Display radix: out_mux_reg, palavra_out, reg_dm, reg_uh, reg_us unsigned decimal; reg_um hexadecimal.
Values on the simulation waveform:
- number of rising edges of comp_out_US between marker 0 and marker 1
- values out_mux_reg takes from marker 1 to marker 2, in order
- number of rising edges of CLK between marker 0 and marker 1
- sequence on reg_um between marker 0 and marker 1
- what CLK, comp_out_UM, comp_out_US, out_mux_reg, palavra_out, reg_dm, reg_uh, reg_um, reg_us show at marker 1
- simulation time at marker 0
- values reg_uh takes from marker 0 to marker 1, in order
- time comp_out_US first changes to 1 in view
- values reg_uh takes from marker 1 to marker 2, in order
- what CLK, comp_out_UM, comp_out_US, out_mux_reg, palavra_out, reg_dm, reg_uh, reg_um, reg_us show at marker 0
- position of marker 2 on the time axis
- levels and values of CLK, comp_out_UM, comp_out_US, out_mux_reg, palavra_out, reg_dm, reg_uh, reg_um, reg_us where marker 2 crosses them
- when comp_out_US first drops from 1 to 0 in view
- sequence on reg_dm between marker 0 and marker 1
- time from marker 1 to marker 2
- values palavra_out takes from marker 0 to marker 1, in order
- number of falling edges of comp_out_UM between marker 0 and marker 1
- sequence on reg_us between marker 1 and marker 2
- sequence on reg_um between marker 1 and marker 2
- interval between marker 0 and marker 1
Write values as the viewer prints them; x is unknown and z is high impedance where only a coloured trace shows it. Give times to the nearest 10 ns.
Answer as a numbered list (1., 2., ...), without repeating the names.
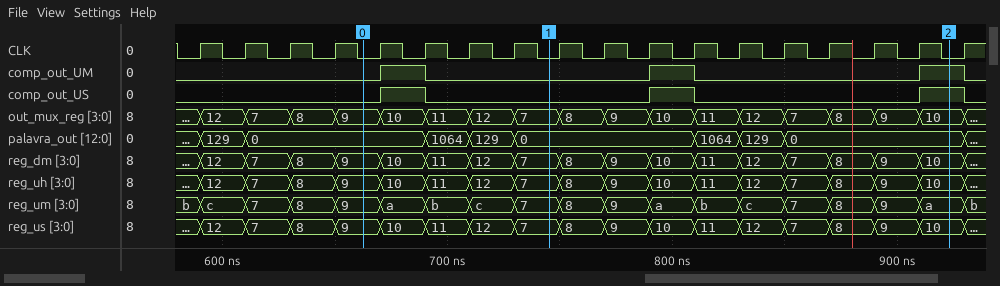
1. 1
2. 7, 8, 9, 10, 11, 12, 7, 8, 9, 10
3. 4
4. 9, a, b, c, 7
5. CLK=0, comp_out_UM=0, comp_out_US=0, out_mux_reg=7, palavra_out=0, reg_dm=7, reg_uh=7, reg_um=7, reg_us=7
6. 660 ns
7. 9, 10, 11, 12, 7
8. 670 ns
9. 7, 8, 9, 10, 11, 12, 7, 8, 9, 10
10. CLK=0, comp_out_UM=0, comp_out_US=0, out_mux_reg=9, palavra_out=0, reg_dm=9, reg_uh=9, reg_um=9, reg_us=9
11. 920 ns
12. CLK=0, comp_out_UM=1, comp_out_US=1, out_mux_reg=10, palavra_out=0, reg_dm=10, reg_uh=10, reg_um=a, reg_us=10
13. 690 ns
14. 9, 10, 11, 12, 7
15. 180 ns
16. 0, 1064, 129, 0
17. 1
18. 7, 8, 9, 10, 11, 12, 7, 8, 9, 10
19. 7, 8, 9, a, b, c, 7, 8, 9, a
20. 80 ns
